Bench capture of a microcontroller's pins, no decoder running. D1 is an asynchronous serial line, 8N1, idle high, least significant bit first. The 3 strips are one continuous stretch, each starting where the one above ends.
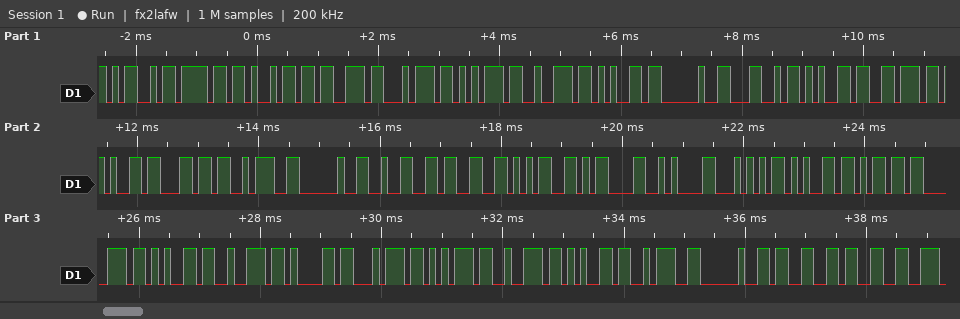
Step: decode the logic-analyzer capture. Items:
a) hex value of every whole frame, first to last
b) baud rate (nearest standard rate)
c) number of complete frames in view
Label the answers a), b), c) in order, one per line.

a) 4D 6F 69 73 74 75 72 65 20 4C 65 76 65 6C 3A 20 32 33 35 0D 0A 54 65 6D 70 65 72 61 74 75 72 65 3A 20 33 33
b) 9600 baud
c) 36
